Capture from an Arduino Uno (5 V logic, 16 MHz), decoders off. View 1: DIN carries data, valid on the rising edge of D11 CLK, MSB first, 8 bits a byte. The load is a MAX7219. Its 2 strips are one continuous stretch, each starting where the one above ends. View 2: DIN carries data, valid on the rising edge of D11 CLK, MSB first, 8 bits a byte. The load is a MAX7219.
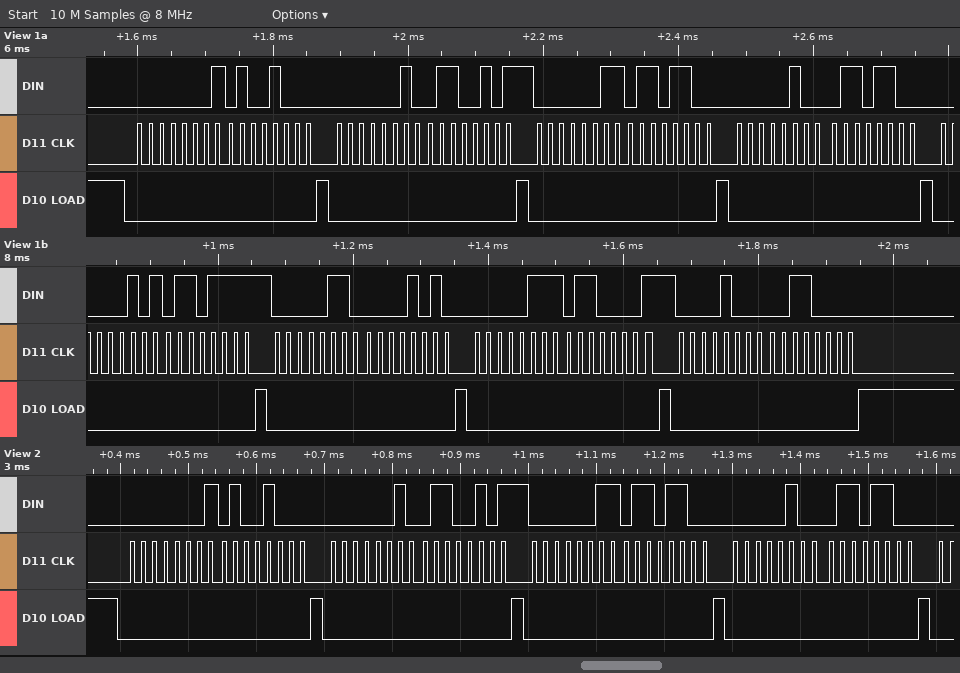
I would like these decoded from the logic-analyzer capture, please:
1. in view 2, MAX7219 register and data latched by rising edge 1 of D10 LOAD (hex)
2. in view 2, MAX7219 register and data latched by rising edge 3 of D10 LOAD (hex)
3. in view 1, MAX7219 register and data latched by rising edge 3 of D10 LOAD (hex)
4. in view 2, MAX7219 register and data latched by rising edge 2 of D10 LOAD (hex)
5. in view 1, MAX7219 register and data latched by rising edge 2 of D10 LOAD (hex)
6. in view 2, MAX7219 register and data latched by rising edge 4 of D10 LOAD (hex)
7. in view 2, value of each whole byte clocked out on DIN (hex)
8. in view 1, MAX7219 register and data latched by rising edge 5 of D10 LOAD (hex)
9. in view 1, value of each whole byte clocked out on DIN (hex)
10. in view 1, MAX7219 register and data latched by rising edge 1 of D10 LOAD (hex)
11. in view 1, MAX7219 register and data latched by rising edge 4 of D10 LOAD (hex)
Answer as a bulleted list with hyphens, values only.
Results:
- register 0x1, data 0x48
- register 0x3, data 0x6C
- register 0x3, data 0x6C
- register 0x2, data 0x65
- register 0x2, data 0x65
- register 0x4, data 0x6C
- 01 48 02 65 03 6C 04 6C
- register 0x5, data 0x6F
- 01 48 02 65 03 6C 04 6C 05 6F 06 0A 07 61 08 30
- register 0x1, data 0x48
- register 0x4, data 0x6C
